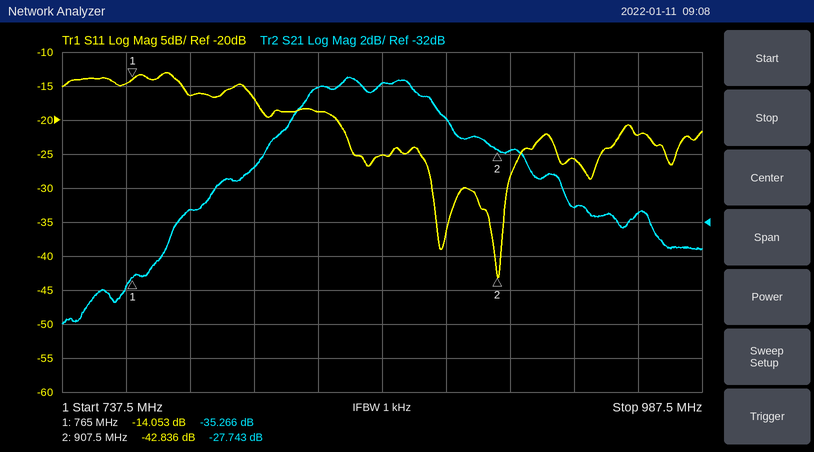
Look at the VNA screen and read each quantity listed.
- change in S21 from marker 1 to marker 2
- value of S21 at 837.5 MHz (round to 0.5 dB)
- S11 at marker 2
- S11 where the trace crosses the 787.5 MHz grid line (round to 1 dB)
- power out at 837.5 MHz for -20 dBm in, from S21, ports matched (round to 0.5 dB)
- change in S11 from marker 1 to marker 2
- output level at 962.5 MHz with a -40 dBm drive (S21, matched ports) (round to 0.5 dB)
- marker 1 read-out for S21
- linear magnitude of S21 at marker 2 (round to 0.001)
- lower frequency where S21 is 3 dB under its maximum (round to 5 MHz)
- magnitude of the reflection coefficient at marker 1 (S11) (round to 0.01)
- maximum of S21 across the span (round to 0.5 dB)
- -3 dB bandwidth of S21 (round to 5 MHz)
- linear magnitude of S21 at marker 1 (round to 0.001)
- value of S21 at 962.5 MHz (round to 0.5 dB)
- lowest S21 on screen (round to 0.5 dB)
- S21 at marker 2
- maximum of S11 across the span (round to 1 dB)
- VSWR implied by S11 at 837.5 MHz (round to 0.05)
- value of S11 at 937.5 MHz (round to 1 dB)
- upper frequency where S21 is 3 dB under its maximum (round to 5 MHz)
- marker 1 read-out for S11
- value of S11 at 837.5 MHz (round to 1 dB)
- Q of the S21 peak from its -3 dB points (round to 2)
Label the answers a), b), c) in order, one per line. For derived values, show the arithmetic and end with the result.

a) -27.743 − (-35.266) = 7.523 dB
b) -24.0 dB
c) -42.836 dB
d) -16 dB
e) -20 dBm + (-24.0 dB) = -44.0 dBm
f) -42.836 − (-14.053) = -28.783 dB
g) -40 dBm + (-31.5 dB) = -71.5 dBm
h) -35.266 dB
i) 10^(-27.743/20) ≈ 0.041
j) 825 MHz
k) 10^(-14.053/20) ≈ 0.20
l) -23.5 dB
m) 890 MHz − 825 MHz = 65 MHz
n) 10^(-35.266/20) ≈ 0.017
o) -31.5 dB
p) -38.0 dB
q) -27.743 dB
r) -13 dB
s) |Γ| = 10^(-19/20) = 0.1122; VSWR = (1 + 0.1122)/(1 − 0.1122) ≈ 1.25
t) -26 dB
u) 890 MHz
v) -14.053 dB
w) -19 dB
x) 857.5 MHz / 65 MHz ≈ 13.2, so 14 to the nearest 2
